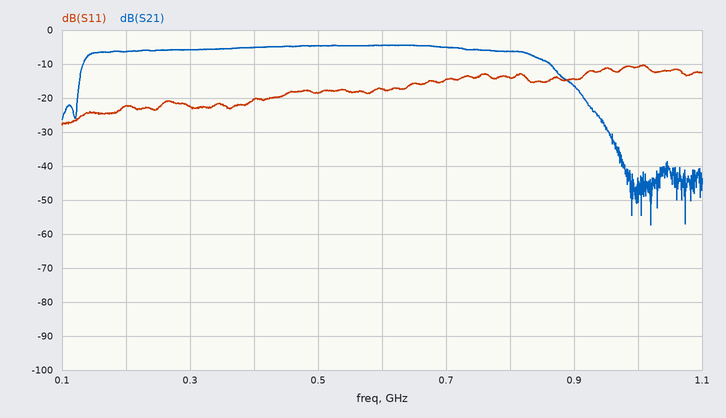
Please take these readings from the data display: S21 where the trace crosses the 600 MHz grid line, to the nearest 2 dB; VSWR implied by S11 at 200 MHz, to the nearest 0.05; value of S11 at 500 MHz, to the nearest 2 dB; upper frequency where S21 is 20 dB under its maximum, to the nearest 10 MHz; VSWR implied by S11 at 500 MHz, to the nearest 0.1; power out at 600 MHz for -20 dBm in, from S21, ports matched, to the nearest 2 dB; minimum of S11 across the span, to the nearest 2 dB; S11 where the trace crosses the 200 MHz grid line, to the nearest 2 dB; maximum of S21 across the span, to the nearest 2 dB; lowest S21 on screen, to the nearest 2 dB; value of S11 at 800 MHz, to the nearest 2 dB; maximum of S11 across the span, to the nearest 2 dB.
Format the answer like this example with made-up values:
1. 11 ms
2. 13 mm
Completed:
1. -4 dB
2. 1.15
3. -18 dB
4. 930 MHz
5. 1.3
6. -24 dBm
7. -28 dB
8. -22 dB
9. -4 dB
10. -58 dB
11. -14 dB
12. -10 dB
